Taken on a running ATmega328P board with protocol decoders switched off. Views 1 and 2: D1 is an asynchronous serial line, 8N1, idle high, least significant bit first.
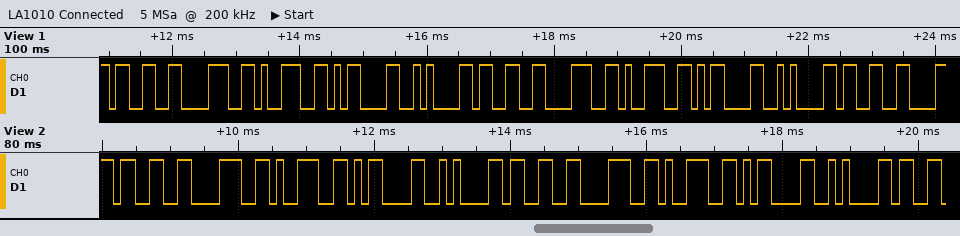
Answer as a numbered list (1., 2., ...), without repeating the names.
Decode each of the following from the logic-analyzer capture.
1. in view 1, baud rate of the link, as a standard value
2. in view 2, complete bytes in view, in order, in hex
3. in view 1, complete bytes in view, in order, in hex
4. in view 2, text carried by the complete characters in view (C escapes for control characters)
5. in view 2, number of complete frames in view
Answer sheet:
1. 9600 baud
2. 33 38 39 0D 0A 33 38 39 0D 0A
3. 33 38 39 0D 0A 33 38 39 0D 0A 33
4. "389\r\n389\r\n"
5. 10
